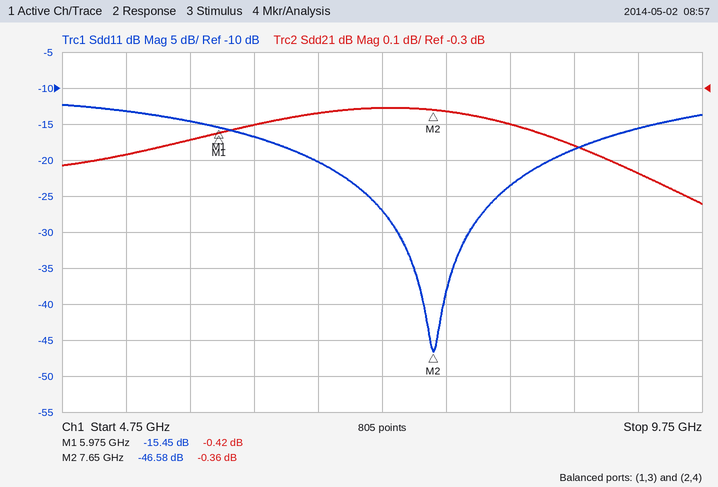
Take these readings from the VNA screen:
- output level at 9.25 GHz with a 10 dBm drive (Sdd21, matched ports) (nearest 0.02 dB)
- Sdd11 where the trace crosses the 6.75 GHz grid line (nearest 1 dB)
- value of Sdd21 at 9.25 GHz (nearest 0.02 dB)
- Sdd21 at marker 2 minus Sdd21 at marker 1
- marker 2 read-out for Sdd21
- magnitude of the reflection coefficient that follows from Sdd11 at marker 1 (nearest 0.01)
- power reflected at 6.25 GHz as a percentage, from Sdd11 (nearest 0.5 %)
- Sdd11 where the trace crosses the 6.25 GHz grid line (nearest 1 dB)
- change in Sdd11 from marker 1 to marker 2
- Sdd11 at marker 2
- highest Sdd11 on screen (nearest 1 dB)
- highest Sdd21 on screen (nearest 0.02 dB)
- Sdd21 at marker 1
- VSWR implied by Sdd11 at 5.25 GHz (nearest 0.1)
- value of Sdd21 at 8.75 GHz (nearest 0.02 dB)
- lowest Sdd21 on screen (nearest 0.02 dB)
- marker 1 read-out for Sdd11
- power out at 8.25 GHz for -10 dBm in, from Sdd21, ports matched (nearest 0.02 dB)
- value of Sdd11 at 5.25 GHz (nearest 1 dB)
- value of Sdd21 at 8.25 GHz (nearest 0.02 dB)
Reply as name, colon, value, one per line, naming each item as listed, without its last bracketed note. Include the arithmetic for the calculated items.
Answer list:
output level at 9.25 GHz with a 10 dBm drive (Sdd21, matched ports): 10 dBm + (-0.54 dB) = 9.46 dBm
Sdd11 where the trace crosses the 6.75 GHz grid line: -20 dB
value of Sdd21 at 9.25 GHz: -0.54 dB
Sdd21 at marker 2 minus Sdd21 at marker 1: -0.36 − (-0.42) = 0.06 dB
marker 2 read-out for Sdd21: -0.36 dB
magnitude of the reflection coefficient that follows from Sdd11 at marker 1: 10^(-15.45/20) ≈ 0.17
power reflected at 6.25 GHz as a percentage, from Sdd11: 10^(-17/10) ≈ 2.0 %
Sdd11 where the trace crosses the 6.25 GHz grid line: -17 dB
change in Sdd11 from marker 1 to marker 2: -46.58 − (-15.45) = -31.13 dB
Sdd11 at marker 2: -46.58 dB
highest Sdd11 on screen: -12 dB
highest Sdd21 on screen: -0.36 dB
Sdd21 at marker 1: -0.42 dB
VSWR implied by Sdd11 at 5.25 GHz: |Γ| = 10^(-13/20) = 0.2239; VSWR = (1 + 0.2239)/(1 − 0.2239) ≈ 1.6
value of Sdd21 at 8.75 GHz: -0.46 dB
lowest Sdd21 on screen: -0.62 dB
marker 1 read-out for Sdd11: -15.45 dB
power out at 8.25 GHz for -10 dBm in, from Sdd21, ports matched: -10 dBm + (-0.40 dB) = -10.40 dBm
value of Sdd11 at 5.25 GHz: -13 dB
value of Sdd21 at 8.25 GHz: -0.40 dB
